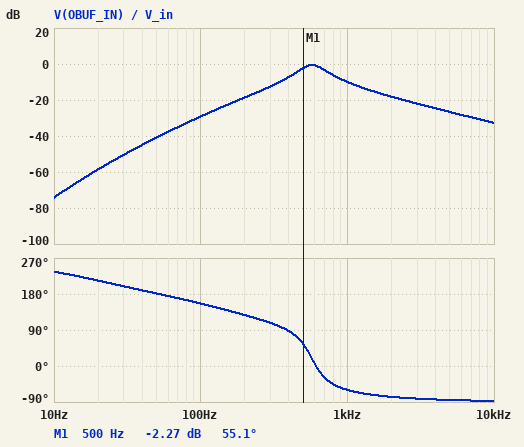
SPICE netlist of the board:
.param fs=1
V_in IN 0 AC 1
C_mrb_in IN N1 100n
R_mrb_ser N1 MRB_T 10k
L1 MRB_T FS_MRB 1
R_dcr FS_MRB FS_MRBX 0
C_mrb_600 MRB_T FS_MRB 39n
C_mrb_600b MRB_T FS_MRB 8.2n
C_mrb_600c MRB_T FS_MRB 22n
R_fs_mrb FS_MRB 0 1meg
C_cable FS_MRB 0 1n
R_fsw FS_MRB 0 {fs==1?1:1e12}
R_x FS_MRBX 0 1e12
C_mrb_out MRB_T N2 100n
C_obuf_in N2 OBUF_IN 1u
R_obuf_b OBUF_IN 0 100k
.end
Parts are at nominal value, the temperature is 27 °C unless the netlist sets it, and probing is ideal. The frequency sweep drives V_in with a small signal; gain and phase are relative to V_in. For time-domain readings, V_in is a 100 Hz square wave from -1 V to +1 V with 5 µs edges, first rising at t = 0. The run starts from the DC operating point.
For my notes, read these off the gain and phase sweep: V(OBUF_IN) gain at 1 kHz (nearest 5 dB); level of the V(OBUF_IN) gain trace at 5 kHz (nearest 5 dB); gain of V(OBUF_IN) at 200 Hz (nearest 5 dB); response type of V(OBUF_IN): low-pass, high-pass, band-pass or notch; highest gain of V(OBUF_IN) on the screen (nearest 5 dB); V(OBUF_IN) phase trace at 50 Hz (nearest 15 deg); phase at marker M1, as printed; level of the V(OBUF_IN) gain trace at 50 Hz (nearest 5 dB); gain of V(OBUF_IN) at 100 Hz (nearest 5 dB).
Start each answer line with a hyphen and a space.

- -10 dB
- -25 dB
- -20 dB
- band-pass
- 0 dB
- 180 deg
- 55.1 deg
- -40 dB
- -30 dB
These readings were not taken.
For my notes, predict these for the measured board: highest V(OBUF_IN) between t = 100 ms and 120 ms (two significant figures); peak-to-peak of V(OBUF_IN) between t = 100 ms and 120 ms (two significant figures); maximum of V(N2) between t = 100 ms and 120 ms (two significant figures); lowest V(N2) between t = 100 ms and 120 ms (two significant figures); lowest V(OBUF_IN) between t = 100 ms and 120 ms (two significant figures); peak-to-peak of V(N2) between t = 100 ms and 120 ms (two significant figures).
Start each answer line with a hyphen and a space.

- 460 mV
- 920 mV
- 460 mV
- -460 mV
- -460 mV
- 920 mV
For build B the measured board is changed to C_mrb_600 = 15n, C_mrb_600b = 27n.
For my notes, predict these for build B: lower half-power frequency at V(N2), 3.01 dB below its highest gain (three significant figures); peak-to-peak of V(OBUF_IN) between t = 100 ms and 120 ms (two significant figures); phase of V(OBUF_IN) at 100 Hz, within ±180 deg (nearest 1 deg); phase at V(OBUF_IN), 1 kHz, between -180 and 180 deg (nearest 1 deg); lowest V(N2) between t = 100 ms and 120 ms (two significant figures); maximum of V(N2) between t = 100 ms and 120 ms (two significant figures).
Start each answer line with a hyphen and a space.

- 485 Hz
- 940 mV
- 156 deg
- -57 deg
- -470 mV
- 470 mV
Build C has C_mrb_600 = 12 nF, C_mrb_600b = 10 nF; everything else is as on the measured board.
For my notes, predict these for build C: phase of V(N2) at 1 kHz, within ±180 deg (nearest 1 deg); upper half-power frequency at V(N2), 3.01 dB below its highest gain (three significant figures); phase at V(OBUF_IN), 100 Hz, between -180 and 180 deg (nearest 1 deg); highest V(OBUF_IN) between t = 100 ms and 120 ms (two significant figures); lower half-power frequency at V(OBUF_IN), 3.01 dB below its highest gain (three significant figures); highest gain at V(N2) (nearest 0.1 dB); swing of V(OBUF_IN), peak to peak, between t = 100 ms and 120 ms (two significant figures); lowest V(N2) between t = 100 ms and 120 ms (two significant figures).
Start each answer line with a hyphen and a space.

- -41 deg
- 936 Hz
- 156 deg
- 570 mV
- 557 Hz
- -0.7 dB
- 1.1 V
- -570 mV
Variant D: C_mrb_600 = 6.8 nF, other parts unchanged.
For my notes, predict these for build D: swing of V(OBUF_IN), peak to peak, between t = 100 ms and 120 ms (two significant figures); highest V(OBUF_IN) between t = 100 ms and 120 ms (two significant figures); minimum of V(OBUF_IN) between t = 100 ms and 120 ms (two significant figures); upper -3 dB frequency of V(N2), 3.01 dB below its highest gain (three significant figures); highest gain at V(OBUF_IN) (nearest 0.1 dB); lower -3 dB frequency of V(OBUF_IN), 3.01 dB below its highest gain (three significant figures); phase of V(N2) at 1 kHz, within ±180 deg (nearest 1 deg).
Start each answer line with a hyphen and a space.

- 1.2 V
- 610 mV
- -610 mV
- 1.05 kHz
- -0.7 dB
- 592 Hz
- -30 deg
